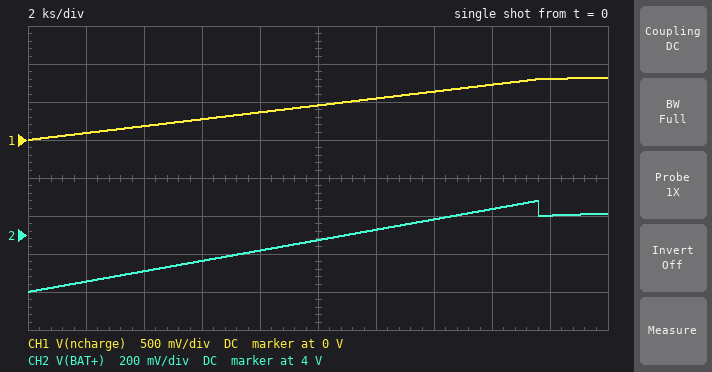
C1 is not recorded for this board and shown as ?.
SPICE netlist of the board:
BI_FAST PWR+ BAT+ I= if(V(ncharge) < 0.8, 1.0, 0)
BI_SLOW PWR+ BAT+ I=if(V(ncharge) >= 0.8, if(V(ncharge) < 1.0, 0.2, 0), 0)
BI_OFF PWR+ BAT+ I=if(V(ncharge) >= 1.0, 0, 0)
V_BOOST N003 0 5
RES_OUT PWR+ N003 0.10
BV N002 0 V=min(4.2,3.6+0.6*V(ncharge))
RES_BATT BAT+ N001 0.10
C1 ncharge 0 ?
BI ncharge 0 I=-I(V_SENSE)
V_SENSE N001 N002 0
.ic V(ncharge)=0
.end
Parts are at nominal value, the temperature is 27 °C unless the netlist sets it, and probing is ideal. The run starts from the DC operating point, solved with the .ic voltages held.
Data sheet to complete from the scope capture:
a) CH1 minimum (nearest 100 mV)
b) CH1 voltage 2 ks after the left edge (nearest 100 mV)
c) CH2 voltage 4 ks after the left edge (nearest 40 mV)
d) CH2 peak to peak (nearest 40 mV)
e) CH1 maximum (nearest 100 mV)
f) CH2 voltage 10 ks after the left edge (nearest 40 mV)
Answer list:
0 V
100 mV
3.80 V
480 mV
800 mV
3.96 V
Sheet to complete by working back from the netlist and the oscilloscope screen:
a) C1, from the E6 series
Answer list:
22 kF
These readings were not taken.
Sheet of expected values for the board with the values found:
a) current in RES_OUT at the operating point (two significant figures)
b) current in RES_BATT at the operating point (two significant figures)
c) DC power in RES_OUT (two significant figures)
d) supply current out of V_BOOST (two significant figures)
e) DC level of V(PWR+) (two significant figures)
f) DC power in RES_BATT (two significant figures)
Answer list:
1.0 A
1.0 A
100 mW
1.0 A
4.9 V
100 mW
